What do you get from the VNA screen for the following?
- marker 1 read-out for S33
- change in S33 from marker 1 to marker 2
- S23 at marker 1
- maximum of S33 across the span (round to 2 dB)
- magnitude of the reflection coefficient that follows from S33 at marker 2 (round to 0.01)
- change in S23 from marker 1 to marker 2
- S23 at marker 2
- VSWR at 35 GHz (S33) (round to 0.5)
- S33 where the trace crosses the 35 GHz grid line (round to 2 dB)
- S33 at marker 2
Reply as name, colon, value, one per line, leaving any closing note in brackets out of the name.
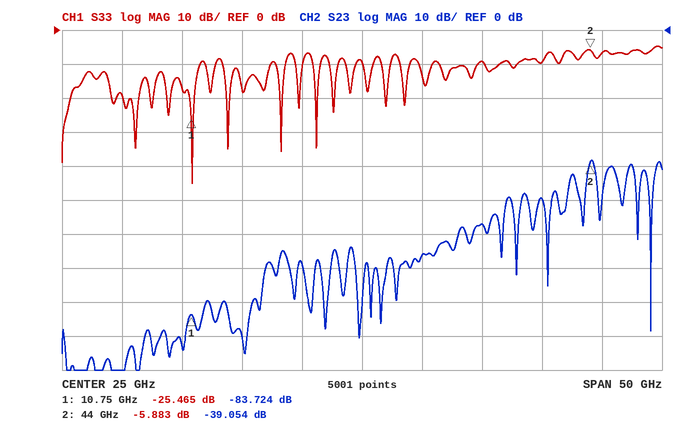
marker 1 read-out for S33: -25.465 dB
change in S33 from marker 1 to marker 2: 19.582 dB
S23 at marker 1: -83.724 dB
maximum of S33 across the span: -4 dB
magnitude of the reflection coefficient that follows from S33 at marker 2: 0.51
change in S23 from marker 1 to marker 2: 44.670 dB
S23 at marker 2: -39.054 dB
VSWR at 35 GHz (S33): 2.0
S33 where the trace crosses the 35 GHz grid line: -10 dB
S33 at marker 2: -5.883 dB
